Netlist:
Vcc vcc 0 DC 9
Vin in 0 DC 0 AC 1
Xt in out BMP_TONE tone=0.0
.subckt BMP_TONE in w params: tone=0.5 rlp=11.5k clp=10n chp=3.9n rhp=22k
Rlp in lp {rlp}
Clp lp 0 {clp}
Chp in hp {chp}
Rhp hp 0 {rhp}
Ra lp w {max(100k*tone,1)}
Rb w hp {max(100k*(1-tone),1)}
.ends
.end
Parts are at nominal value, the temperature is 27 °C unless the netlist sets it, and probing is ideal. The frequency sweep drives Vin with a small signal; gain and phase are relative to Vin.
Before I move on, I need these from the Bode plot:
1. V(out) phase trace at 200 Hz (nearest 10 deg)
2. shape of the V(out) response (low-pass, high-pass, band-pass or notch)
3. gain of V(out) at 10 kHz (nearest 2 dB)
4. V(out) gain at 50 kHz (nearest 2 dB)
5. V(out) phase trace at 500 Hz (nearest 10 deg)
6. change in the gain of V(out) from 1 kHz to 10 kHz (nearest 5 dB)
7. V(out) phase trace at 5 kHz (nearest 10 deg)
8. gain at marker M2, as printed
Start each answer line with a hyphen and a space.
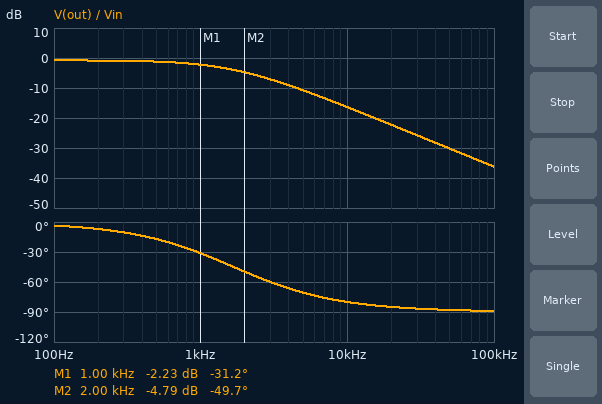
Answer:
- -10 deg
- low-pass
- -16 dB
- -30 dB
- -20 deg
- -15 dB
- -70 deg
- -4.79 dB
